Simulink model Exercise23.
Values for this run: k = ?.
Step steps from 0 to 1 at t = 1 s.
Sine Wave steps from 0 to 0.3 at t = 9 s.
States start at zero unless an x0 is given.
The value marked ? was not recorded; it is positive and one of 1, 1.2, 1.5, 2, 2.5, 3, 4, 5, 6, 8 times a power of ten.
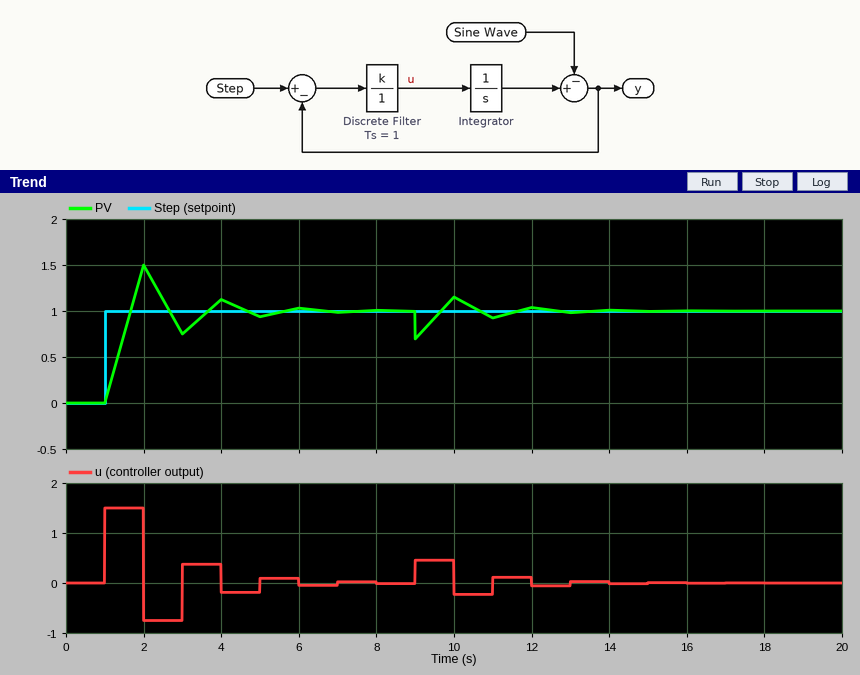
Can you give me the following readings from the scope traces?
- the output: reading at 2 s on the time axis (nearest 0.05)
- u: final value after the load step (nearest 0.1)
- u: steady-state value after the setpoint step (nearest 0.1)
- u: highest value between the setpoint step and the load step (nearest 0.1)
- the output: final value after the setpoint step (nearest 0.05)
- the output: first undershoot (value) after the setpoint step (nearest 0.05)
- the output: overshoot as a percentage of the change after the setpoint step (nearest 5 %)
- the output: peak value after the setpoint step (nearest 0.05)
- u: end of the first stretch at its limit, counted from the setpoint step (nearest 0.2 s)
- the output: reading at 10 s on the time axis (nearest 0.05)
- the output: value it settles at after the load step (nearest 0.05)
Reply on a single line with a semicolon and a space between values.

1.50; 0.0; 0.0; 1.5; 1.00; 0.75; 50 %; 1.50; 1.0 s; 1.15; 1.00
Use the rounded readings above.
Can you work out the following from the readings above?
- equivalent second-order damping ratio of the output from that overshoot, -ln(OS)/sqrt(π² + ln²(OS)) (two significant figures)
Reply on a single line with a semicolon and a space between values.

0.22
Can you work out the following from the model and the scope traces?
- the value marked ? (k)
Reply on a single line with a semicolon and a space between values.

1.5
